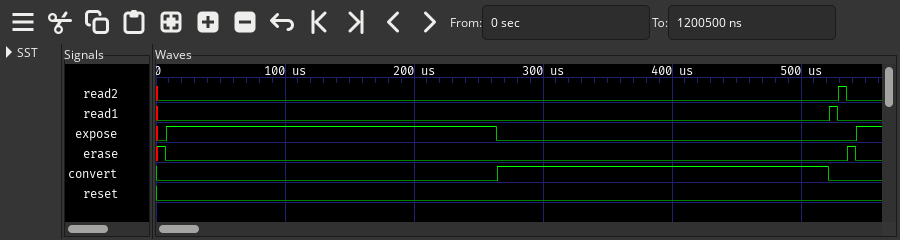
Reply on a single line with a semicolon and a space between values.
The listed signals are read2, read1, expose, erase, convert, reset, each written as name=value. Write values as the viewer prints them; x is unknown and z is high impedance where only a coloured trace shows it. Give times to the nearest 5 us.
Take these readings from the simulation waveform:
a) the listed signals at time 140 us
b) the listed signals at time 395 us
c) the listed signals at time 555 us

read2=0, read1=0, expose=1, erase=0, convert=0, reset=0; read2=0, read1=0, expose=0, erase=0, convert=1, reset=0; read2=0, read1=0, expose=1, erase=0, convert=0, reset=0
